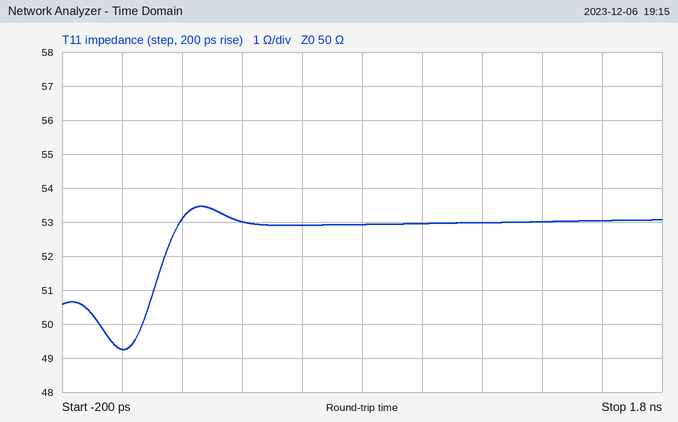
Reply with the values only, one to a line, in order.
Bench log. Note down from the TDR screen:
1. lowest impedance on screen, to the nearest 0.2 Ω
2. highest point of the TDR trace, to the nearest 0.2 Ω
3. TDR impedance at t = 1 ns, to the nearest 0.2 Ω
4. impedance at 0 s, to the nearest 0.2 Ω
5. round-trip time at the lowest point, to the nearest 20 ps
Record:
49.2 Ω
53.4 Ω
53.0 Ω
49.2 Ω
0 ps
